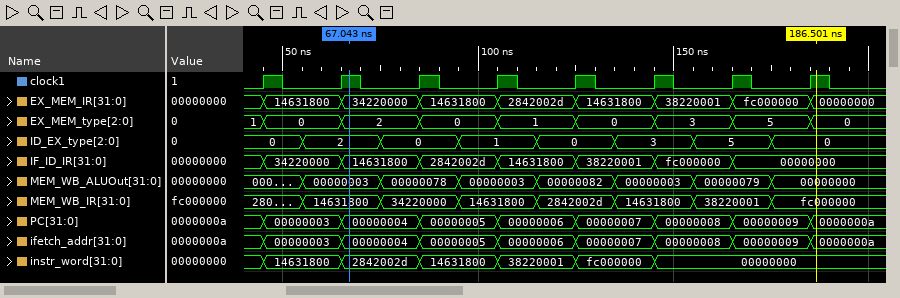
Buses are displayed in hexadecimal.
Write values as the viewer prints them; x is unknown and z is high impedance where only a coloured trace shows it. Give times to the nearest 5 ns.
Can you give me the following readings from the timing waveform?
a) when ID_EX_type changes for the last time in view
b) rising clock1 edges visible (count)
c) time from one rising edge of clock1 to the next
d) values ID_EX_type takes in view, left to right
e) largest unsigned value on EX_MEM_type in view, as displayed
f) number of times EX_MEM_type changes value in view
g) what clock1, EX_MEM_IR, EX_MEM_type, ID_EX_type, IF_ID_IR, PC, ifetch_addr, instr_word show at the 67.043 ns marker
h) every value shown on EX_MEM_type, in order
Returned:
175 ns
8
20 ns
0, 2, 0, 1, 0, 3, 5, 0
5
8
clock1=1, EX_MEM_IR=34220000, EX_MEM_type=2, ID_EX_type=2, IF_ID_IR=14631800, PC=00000004, ifetch_addr=00000004, instr_word=2842002d
1, 0, 2, 0, 1, 0, 3, 5, 0
